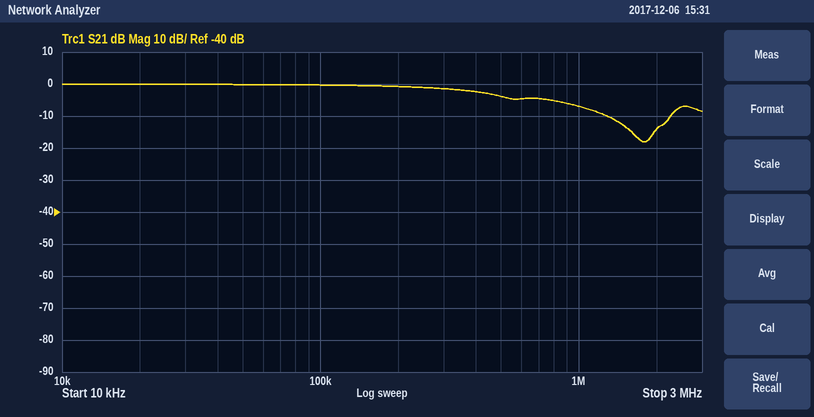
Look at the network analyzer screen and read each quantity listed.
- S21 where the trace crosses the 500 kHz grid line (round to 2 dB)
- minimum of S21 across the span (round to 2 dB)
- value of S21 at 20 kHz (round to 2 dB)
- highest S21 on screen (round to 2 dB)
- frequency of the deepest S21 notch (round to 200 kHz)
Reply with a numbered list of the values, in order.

1. -4 dB
2. -18 dB
3. 0 dB
4. 0 dB
5. 1.8 MHz
